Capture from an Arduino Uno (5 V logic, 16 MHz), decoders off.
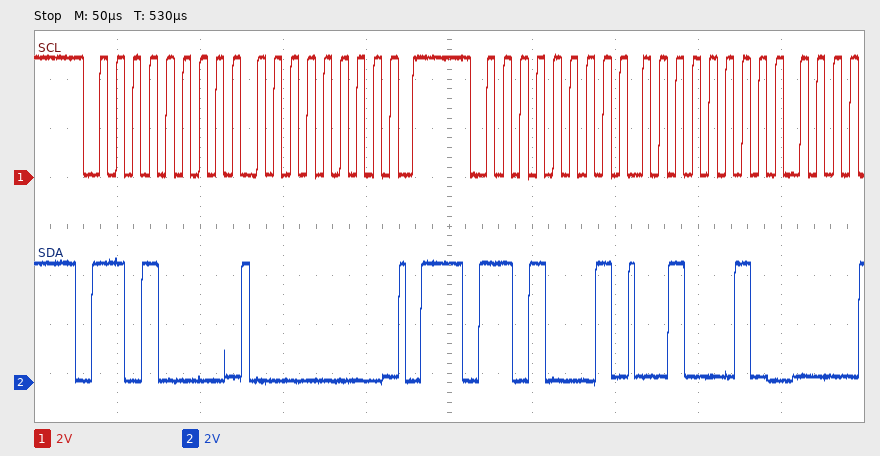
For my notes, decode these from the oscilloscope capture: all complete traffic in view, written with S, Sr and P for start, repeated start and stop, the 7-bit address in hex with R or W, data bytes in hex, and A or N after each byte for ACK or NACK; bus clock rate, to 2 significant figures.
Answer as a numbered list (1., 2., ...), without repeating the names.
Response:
1. S 68W A 00 A P S 68R A 22 A
2. 100 kHz
